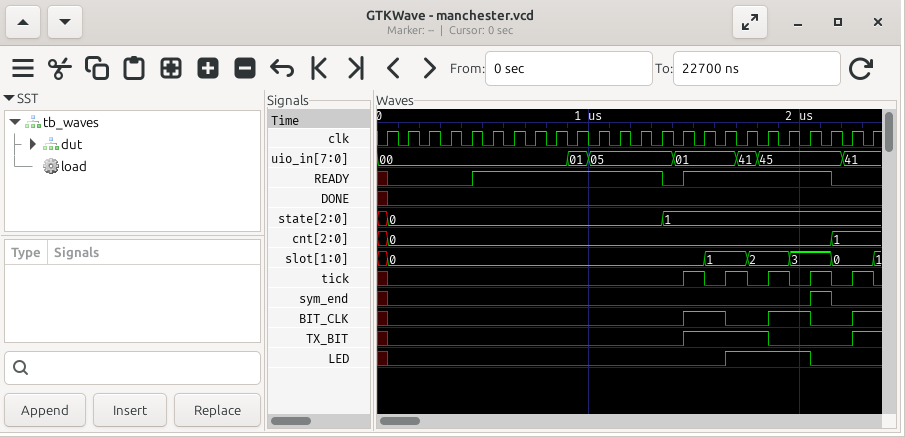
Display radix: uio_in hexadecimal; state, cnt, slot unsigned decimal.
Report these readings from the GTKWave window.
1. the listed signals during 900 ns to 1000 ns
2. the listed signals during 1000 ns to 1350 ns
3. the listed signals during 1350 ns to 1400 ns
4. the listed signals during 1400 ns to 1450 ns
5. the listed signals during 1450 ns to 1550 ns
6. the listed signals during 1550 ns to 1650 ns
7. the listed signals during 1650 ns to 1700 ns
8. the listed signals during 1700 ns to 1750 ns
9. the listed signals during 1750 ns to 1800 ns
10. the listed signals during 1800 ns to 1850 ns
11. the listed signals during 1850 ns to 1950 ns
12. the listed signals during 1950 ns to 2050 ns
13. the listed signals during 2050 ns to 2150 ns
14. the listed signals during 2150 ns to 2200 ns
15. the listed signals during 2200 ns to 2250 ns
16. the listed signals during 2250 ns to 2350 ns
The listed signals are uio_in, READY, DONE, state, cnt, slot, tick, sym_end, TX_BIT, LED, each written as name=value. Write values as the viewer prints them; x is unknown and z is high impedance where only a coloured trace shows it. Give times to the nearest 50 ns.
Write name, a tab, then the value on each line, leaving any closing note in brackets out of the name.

the listed signals during 900 ns to 1000 ns	uio_in=01, READY=1, DONE=0, state=0, cnt=0, slot=0, tick=0, sym_end=0, TX_BIT=0, LED=0
the listed signals during 1000 ns to 1350 ns	uio_in=05, READY=1, DONE=0, state=0, cnt=0, slot=0, tick=0, sym_end=0, TX_BIT=0, LED=0
the listed signals during 1350 ns to 1400 ns	uio_in=05, READY=0, DONE=0, state=1, cnt=0, slot=0, tick=0, sym_end=0, TX_BIT=0, LED=0
the listed signals during 1400 ns to 1450 ns	uio_in=01, READY=0, DONE=0, state=1, cnt=0, slot=0, tick=0, sym_end=0, TX_BIT=0, LED=0
the listed signals during 1450 ns to 1550 ns	uio_in=01, READY=1, DONE=0, state=1, cnt=0, slot=0, tick=1, sym_end=0, TX_BIT=1, LED=0
the listed signals during 1550 ns to 1650 ns	uio_in=01, READY=1, DONE=0, state=1, cnt=0, slot=1, tick=0, sym_end=0, TX_BIT=1, LED=0
the listed signals during 1650 ns to 1700 ns	uio_in=01, READY=1, DONE=0, state=1, cnt=0, slot=1, tick=1, sym_end=0, TX_BIT=1, LED=1
the listed signals during 1700 ns to 1750 ns	uio_in=41, READY=1, DONE=0, state=1, cnt=0, slot=1, tick=1, sym_end=0, TX_BIT=1, LED=1
the listed signals during 1750 ns to 1800 ns	uio_in=41, READY=1, DONE=0, state=1, cnt=0, slot=2, tick=0, sym_end=0, TX_BIT=1, LED=1
the listed signals during 1800 ns to 1850 ns	uio_in=45, READY=1, DONE=0, state=1, cnt=0, slot=2, tick=0, sym_end=0, TX_BIT=1, LED=1
the listed signals during 1850 ns to 1950 ns	uio_in=45, READY=1, DONE=0, state=1, cnt=0, slot=2, tick=1, sym_end=0, TX_BIT=0, LED=1
the listed signals during 1950 ns to 2050 ns	uio_in=45, READY=1, DONE=0, state=1, cnt=0, slot=3, tick=0, sym_end=0, TX_BIT=0, LED=1
the listed signals during 2050 ns to 2150 ns	uio_in=45, READY=1, DONE=0, state=1, cnt=0, slot=3, tick=1, sym_end=1, TX_BIT=0, LED=0
the listed signals during 2150 ns to 2200 ns	uio_in=45, READY=0, DONE=0, state=1, cnt=1, slot=0, tick=0, sym_end=0, TX_BIT=0, LED=0
the listed signals during 2200 ns to 2250 ns	uio_in=41, READY=0, DONE=0, state=1, cnt=1, slot=0, tick=0, sym_end=0, TX_BIT=0, LED=0
the listed signals during 2250 ns to 2350 ns	uio_in=41, READY=0, DONE=0, state=1, cnt=1, slot=0, tick=1, sym_end=0, TX_BIT=1, LED=0
